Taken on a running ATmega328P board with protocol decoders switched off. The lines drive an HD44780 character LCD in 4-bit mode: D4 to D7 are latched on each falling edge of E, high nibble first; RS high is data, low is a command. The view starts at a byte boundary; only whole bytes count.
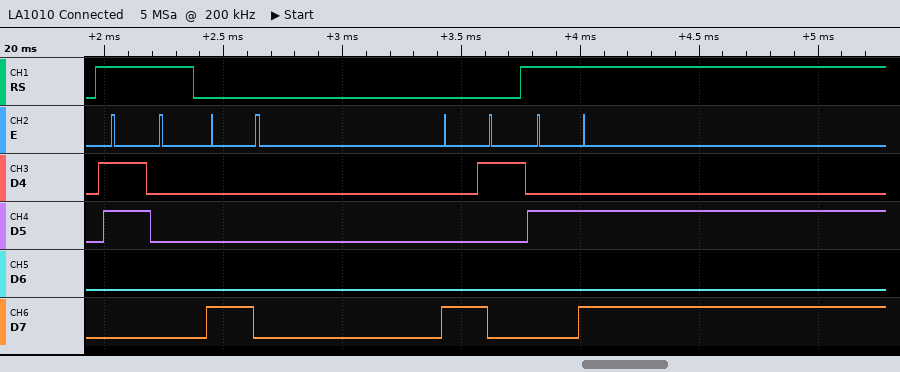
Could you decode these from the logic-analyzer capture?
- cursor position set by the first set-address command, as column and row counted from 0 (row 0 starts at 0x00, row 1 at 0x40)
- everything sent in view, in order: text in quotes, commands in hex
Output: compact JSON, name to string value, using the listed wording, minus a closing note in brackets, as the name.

{"cursor position set by the first set-address command, as column and row counted from 0": "column 0, row 0", "everything sent in view, in order: text in quotes, commands in hex": "\"0\" 0x80 0x81 \"*\""}
